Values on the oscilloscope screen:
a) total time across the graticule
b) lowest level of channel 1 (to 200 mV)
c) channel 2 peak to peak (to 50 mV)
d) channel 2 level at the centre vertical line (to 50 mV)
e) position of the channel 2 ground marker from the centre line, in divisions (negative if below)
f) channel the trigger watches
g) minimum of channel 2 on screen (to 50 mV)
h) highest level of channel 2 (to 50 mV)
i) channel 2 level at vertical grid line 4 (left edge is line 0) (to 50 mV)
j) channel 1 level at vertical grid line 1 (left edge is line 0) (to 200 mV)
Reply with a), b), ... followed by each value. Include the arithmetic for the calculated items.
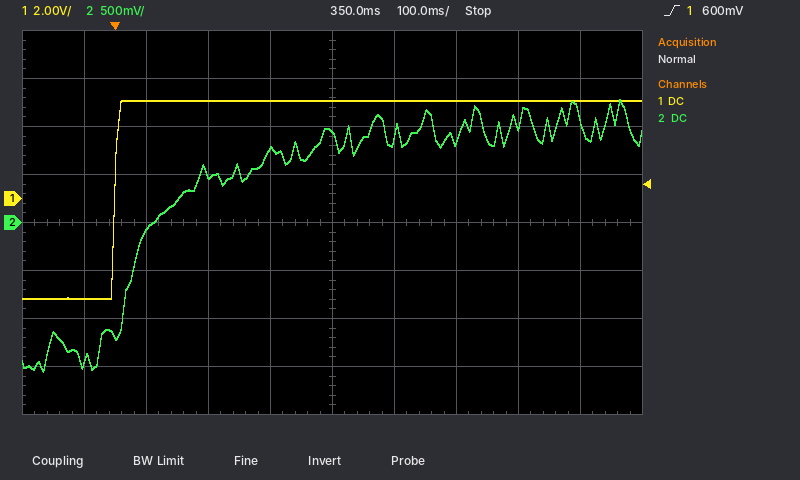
a) 1 s
b) -4.2 V
c) 1.30 V − (-1.55 V) = 2.85 V
d) 950 mV
e) 0.0 div
f) channel 1
g) -1.55 V
h) 1.30 V
i) 750 mV
j) -4.2 V
